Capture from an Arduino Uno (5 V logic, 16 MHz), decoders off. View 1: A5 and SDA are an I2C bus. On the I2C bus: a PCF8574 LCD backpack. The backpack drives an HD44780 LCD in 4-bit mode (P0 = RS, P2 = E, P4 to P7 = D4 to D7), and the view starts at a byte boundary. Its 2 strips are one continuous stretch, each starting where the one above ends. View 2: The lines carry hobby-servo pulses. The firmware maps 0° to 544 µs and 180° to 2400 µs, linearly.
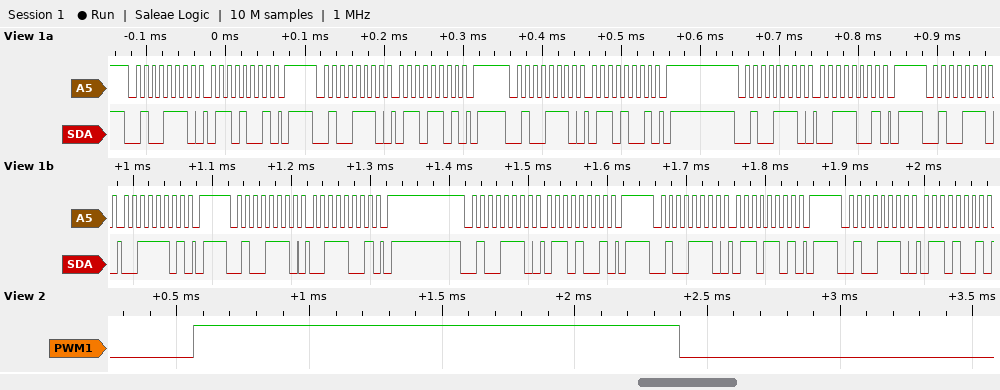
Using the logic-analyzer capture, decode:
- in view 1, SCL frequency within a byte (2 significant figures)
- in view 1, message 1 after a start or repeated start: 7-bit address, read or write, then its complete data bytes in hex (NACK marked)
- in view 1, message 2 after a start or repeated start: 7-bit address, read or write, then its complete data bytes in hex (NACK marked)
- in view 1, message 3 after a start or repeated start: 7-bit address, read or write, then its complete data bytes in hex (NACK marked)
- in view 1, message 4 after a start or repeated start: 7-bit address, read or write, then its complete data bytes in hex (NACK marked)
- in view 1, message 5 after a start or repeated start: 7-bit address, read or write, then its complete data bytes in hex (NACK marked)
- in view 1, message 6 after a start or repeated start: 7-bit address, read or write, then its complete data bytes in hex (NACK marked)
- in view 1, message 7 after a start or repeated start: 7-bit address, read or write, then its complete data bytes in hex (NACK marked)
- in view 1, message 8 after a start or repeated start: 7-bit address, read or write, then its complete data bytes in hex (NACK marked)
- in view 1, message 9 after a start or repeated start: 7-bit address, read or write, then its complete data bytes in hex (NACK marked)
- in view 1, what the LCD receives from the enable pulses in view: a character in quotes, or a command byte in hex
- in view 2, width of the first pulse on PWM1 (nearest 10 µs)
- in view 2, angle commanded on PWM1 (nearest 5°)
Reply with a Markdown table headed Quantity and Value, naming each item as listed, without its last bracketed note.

| Quantity | Value |
|---|---|
| in view 1, SCL frequency within a byte | 100 kHz |
| in view 1, message 1 after a start or repeated start: 7-bit address, read or write, then its complete data bytes in hex | 0x27 write: 69 |
| in view 1, message 2 after a start or repeated start: 7-bit address, read or write, then its complete data bytes in hex | 0x27 write: 6D |
| in view 1, message 3 after a start or repeated start: 7-bit address, read or write, then its complete data bytes in hex | 0x27 write: 69 |
| in view 1, message 4 after a start or repeated start: 7-bit address, read or write, then its complete data bytes in hex | 0x27 write: 39 |
| in view 1, message 5 after a start or repeated start: 7-bit address, read or write, then its complete data bytes in hex | 0x27 write: 3D |
| in view 1, message 6 after a start or repeated start: 7-bit address, read or write, then its complete data bytes in hex | 0x27 write: 39 |
| in view 1, message 7 after a start or repeated start: 7-bit address, read or write, then its complete data bytes in hex | 0x27 write: 69 |
| in view 1, message 8 after a start or repeated start: 7-bit address, read or write, then its complete data bytes in hex | 0x27 write: 6D |
| in view 1, message 9 after a start or repeated start: 7-bit address, read or write, then its complete data bytes in hex | 0x27 write: 69 |
| in view 1, what the LCD receives from the enable pulses in view: a character in quotes, or a command byte in hex | 'c' |
| in view 2, width of the first pulse on PWM1 | 1830 µs |
| in view 2, angle commanded on PWM1 | 125° |
